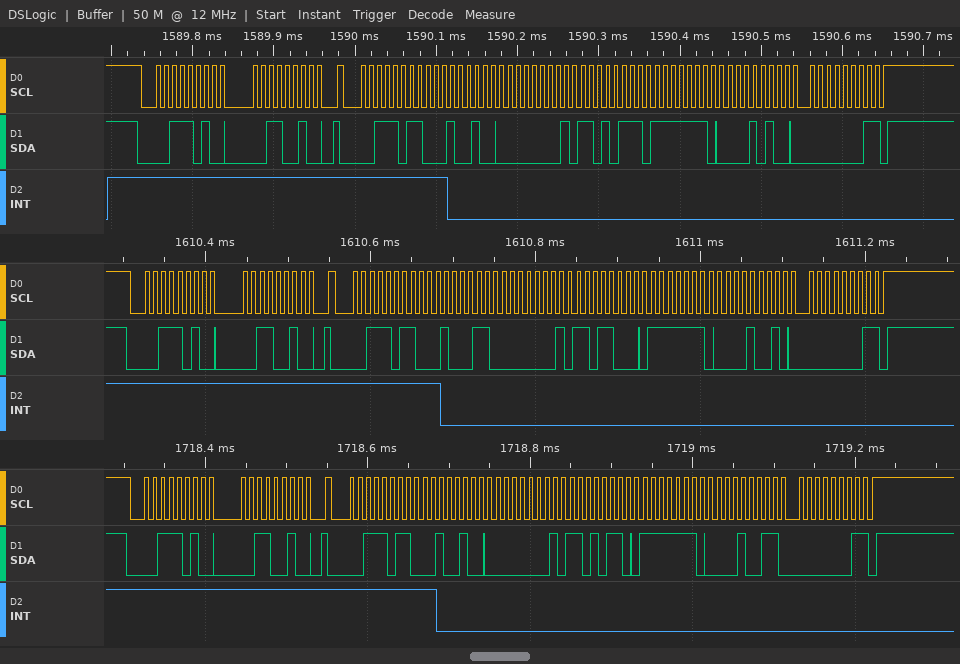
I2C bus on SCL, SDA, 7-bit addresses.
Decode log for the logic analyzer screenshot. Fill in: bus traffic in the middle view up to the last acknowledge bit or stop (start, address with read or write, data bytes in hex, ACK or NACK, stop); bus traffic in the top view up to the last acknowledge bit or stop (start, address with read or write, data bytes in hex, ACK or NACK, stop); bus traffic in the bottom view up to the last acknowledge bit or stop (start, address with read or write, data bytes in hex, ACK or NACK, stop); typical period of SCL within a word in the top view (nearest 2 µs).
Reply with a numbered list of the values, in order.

1. start, address 1D write ACK, 32 ACK, repeated start, address 1D read ACK, 23 ACK, 01 ACK, D8 ACK, FE ACK, 12 ACK, 01 NACK, stop
2. start, address 1D write ACK, 32 ACK, repeated start, address 1D read ACK, 24 ACK, 01 ACK, D7 ACK, FE ACK, 14 ACK, 01 NACK, stop
3. start, address 1D write ACK, 32 ACK, repeated start, address 1D read ACK, 24 ACK, 01 ACK, D6 ACK, FE ACK, 13 ACK, 01 NACK, stop
4. 10 µs
